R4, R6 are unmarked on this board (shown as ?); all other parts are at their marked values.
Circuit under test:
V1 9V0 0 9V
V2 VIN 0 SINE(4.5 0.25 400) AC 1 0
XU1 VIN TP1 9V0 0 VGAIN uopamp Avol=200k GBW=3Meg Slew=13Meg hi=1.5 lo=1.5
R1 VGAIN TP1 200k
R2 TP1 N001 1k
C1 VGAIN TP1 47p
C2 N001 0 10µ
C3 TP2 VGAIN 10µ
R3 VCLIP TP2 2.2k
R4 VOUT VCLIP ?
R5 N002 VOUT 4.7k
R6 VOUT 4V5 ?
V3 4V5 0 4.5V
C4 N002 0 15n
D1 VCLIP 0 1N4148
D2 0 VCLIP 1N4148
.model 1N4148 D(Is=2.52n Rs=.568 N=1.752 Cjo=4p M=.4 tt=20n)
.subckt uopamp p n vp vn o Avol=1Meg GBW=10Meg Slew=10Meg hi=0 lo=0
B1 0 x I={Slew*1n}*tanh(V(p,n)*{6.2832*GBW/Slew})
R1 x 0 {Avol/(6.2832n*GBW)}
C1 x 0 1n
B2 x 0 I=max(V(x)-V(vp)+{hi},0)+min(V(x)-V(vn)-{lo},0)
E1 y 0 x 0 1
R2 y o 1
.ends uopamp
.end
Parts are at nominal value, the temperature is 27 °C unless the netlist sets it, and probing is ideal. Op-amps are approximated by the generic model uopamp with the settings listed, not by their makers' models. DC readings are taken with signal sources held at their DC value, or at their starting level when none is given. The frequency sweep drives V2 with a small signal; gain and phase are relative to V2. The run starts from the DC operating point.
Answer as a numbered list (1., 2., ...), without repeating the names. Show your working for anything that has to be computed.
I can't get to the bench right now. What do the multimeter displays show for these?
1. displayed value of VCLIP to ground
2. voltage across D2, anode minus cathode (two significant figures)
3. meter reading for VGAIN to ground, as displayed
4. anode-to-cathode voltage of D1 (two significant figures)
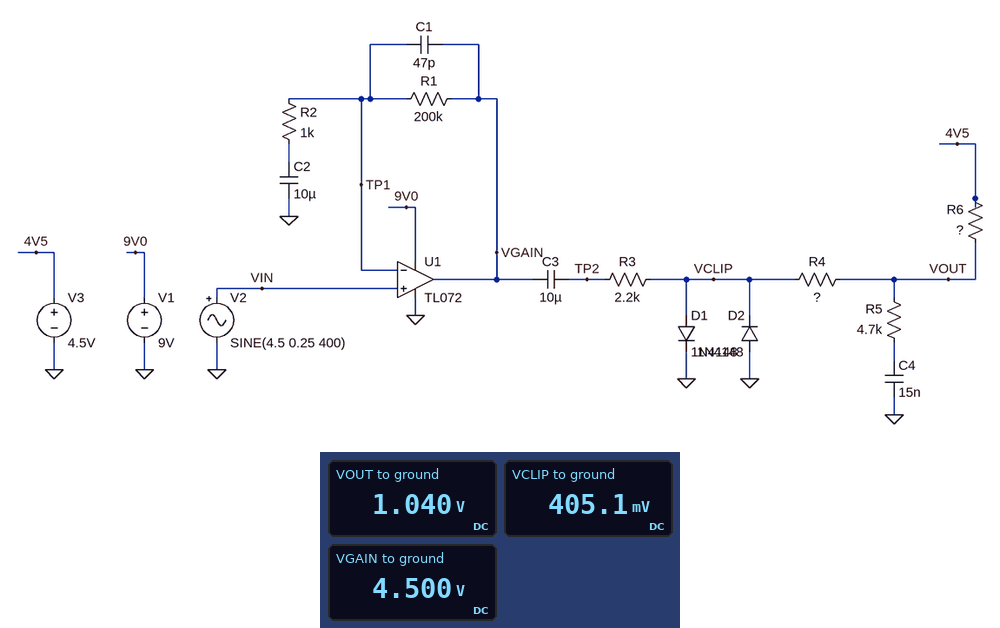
1. 405.1 mV
2. 0 V - 405.1 mV = -410 mV
3. 4.500 V
4. 405.1 mV = 410 mV
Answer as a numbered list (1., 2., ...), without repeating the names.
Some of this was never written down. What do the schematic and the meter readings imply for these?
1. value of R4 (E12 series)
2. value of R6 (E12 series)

1. 33 kΩ
2. 180 kΩ
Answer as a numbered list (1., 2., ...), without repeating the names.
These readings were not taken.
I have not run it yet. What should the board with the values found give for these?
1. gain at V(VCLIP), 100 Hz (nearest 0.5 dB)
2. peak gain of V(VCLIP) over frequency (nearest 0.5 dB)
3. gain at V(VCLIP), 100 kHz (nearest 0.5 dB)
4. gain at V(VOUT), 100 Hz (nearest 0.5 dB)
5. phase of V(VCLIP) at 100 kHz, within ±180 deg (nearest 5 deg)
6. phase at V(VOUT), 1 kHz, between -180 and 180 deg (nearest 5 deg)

1. 40.0 dB
2. 40.0 dB
3. 18.0 dB
4. 38.5 dB
5. -85 deg
6. -55 deg
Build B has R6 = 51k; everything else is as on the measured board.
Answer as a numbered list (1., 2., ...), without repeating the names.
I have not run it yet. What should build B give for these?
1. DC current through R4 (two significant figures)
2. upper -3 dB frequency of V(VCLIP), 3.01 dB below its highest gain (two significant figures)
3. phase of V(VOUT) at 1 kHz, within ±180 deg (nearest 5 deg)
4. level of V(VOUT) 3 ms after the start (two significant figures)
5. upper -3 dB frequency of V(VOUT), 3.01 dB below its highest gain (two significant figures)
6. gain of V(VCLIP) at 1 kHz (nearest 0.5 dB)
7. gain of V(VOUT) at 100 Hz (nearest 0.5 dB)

1. 48 µA
2. 7.9 kHz
3. -50 deg
4. 2.0 V
5. 470 Hz
6. 35.5 dB
7. 31.0 dB
